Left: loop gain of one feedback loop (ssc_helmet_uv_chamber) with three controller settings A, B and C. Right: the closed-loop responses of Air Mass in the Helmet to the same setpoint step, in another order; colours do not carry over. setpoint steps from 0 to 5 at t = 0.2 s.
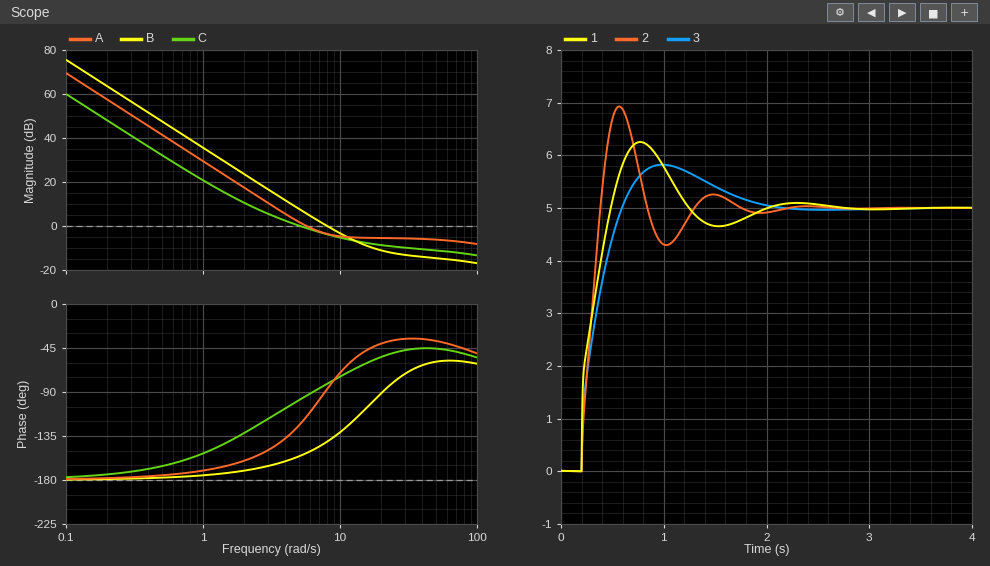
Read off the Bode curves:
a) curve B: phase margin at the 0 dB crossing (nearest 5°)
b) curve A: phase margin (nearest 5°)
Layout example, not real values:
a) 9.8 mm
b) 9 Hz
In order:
a) 40°
b) 65°
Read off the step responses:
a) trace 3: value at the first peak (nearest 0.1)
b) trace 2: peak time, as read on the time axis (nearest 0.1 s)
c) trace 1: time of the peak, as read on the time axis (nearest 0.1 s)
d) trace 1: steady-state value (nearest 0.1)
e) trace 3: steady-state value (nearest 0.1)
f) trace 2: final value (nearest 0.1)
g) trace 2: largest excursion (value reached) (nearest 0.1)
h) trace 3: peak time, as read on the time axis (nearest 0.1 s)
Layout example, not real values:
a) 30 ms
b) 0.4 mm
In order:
a) 5.8
b) 0.6 s
c) 0.8 s
d) 5.0
e) 5.0
f) 5.0
g) 6.9
h) 1.0 s
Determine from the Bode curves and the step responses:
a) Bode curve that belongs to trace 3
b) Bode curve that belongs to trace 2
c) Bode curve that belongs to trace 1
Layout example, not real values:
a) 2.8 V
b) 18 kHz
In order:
a) C
b) B
c) A
